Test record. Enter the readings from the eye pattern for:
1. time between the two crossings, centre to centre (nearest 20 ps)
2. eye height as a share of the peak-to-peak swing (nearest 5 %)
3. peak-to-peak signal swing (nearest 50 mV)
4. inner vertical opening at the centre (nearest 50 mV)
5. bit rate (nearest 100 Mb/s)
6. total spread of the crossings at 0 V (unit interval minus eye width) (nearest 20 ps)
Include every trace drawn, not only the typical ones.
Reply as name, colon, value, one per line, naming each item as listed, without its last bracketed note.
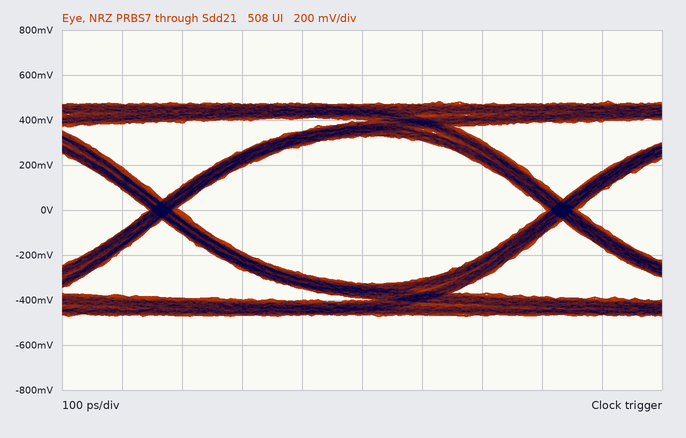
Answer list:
time between the two crossings, centre to centre: 660 ps
eye height as a share of the peak-to-peak swing: 70 %
peak-to-peak signal swing: 950 mV
inner vertical opening at the centre: 650 mV
bit rate: 1.5 Gb/s
total spread of the crossings at 0 V (unit interval minus eye width): 60 ps
